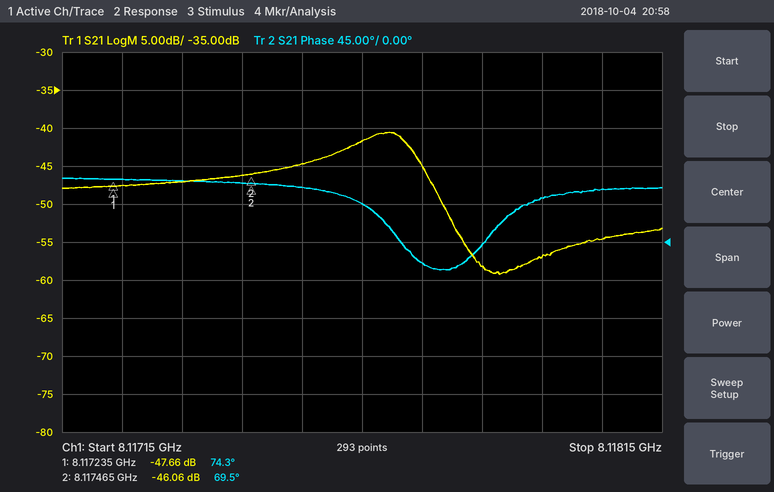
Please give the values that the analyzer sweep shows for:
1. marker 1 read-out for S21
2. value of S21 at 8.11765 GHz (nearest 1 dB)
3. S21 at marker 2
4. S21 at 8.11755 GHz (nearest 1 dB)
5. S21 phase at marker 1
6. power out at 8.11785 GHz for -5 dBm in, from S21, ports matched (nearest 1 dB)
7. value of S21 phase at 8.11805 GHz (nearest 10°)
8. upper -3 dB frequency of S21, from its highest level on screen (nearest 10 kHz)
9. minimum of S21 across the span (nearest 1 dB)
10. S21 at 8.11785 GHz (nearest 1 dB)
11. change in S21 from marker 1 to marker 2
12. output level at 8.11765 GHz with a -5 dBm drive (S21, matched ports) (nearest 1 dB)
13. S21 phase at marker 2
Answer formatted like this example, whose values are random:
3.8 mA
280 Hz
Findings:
-47.66 dB
-42 dB
-46.06 dB
-45 dB
74.3°
-63 dBm
60°
8.11774 GHz
-59 dB
-58 dB
1.60 dB
-47 dBm
69.5°
